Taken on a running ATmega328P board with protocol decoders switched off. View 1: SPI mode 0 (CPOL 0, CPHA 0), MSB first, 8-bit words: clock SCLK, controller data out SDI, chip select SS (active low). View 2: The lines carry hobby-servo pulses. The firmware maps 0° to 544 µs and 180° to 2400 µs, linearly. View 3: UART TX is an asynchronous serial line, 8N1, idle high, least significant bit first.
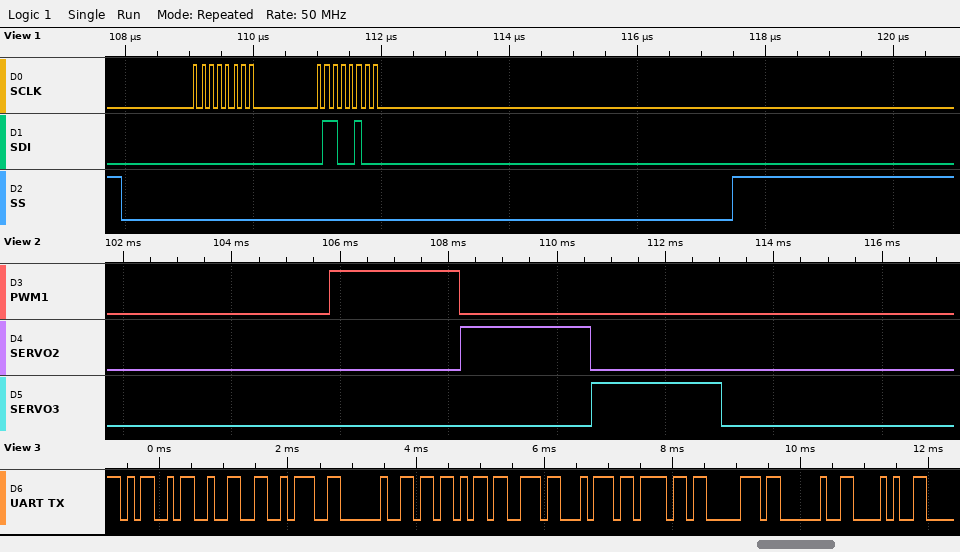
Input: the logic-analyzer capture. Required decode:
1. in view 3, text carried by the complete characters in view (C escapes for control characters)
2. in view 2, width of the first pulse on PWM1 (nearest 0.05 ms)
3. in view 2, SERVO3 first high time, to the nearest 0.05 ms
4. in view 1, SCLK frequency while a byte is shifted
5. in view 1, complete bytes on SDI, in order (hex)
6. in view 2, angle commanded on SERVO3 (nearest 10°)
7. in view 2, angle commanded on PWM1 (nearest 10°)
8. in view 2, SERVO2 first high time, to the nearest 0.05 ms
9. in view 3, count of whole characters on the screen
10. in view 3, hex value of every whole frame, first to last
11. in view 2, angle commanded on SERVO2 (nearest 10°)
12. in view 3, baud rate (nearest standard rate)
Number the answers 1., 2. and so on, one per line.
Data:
1. "M2: [stop ("
2. 2.40 ms
3. 2.40 ms
4. 8 MHz
5. 00 64
6. 180°
7. 180°
8. 2.40 ms
9. 11
10. 4D 32 3A 20 5B 73 74 6F 70 20 28
11. 180°
12. 9600 baud
